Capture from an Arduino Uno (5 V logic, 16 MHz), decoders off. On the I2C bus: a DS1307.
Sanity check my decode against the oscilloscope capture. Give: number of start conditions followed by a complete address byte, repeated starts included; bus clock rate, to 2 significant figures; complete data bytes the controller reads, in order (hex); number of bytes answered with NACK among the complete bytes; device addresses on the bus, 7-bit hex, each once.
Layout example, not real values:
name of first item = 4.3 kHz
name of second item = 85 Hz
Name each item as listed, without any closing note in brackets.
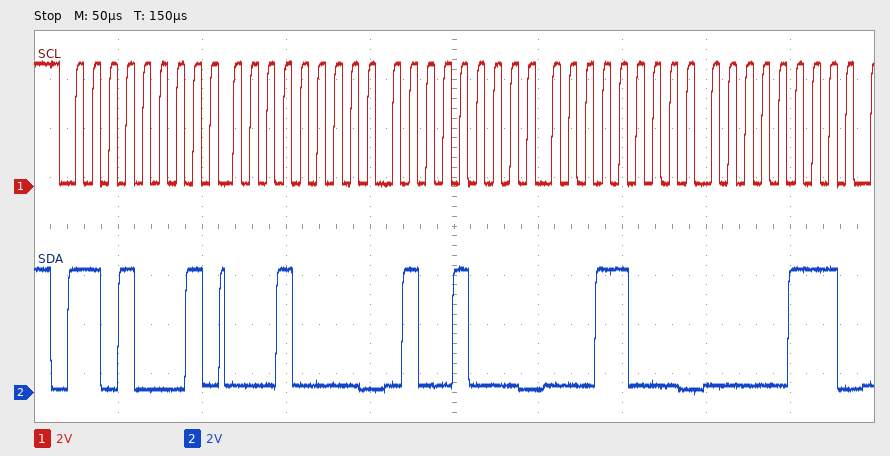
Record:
number of start conditions followed by a complete address byte, repeated starts included = 1
bus clock rate, to 2 significant figures = 100 kHz
complete data bytes the controller reads, in order = 10 48 18 07
number of bytes answered with NACK among the complete bytes = 0
device addresses on the bus, 7-bit hex, each once = 0x68
